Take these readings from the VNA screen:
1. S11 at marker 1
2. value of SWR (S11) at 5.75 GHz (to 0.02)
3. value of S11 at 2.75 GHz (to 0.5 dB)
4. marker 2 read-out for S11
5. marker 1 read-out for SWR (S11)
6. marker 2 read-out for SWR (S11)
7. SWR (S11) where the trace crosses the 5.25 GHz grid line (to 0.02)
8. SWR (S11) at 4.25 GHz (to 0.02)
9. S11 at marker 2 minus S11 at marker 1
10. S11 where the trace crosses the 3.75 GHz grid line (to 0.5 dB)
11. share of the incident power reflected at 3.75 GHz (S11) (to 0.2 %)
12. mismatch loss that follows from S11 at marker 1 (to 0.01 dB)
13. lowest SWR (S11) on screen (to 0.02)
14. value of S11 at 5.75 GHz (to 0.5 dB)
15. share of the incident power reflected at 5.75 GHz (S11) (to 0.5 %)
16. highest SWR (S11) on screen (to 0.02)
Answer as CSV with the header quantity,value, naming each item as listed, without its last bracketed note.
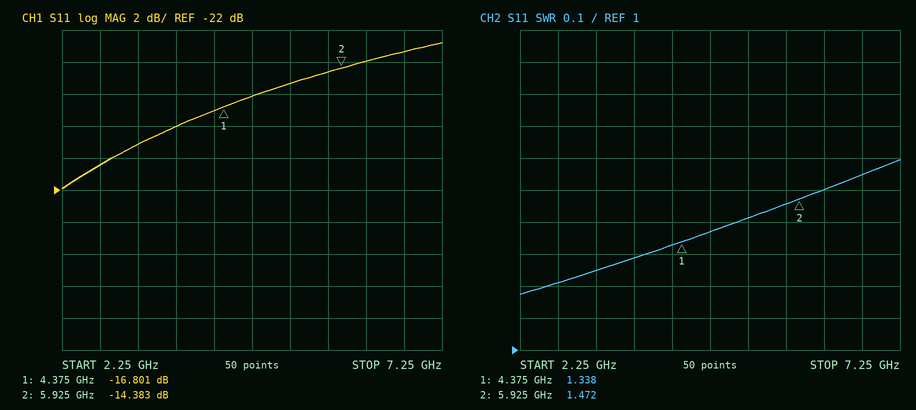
quantity,value
S11 at marker 1,-16.801 dB
value of SWR (S11) at 5.75 GHz,1.46
value of S11 at 2.75 GHz,-20.5 dB
marker 2 read-out for S11,-14.383 dB
marker 1 read-out for SWR,1.338
marker 2 read-out for SWR,1.472
SWR (S11) where the trace crosses the 5.25 GHz grid line,1.42
SWR (S11) at 4.25 GHz,1.32
S11 at marker 2 minus S11 at marker 1,2.418 dB
S11 where the trace crosses the 3.75 GHz grid line,-18.0 dB
share of the incident power reflected at 3.75 GHz (S11),1.6 %
mismatch loss that follows from S11 at marker 1,0.09 dB
lowest SWR (S11) on screen,1.18
value of S11 at 5.75 GHz,-14.5 dB
share of the incident power reflected at 5.75 GHz (S11),3.5 %
highest SWR (S11) on screen,1.60
